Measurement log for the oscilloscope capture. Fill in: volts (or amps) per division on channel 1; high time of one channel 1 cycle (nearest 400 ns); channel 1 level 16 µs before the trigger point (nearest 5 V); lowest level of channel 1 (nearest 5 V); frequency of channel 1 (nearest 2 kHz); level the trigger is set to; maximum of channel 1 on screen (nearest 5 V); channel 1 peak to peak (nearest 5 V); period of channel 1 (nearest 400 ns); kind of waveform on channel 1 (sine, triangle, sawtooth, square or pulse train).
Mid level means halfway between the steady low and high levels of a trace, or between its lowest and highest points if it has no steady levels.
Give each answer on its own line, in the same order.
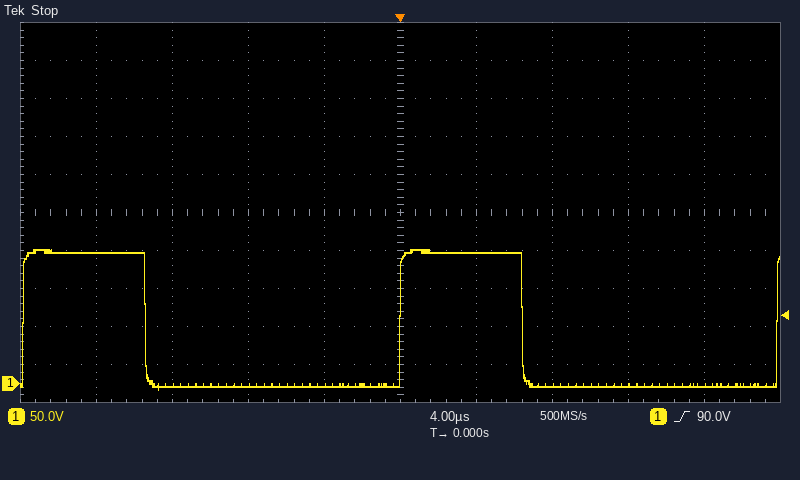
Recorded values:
50 V
6.4 µs
170 V
-10 V
50 kHz
90.0 V
175 V
185 V
20.0 µs
pulse train
